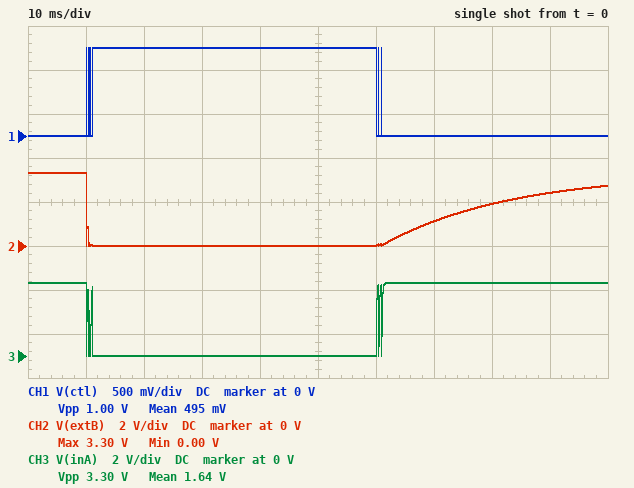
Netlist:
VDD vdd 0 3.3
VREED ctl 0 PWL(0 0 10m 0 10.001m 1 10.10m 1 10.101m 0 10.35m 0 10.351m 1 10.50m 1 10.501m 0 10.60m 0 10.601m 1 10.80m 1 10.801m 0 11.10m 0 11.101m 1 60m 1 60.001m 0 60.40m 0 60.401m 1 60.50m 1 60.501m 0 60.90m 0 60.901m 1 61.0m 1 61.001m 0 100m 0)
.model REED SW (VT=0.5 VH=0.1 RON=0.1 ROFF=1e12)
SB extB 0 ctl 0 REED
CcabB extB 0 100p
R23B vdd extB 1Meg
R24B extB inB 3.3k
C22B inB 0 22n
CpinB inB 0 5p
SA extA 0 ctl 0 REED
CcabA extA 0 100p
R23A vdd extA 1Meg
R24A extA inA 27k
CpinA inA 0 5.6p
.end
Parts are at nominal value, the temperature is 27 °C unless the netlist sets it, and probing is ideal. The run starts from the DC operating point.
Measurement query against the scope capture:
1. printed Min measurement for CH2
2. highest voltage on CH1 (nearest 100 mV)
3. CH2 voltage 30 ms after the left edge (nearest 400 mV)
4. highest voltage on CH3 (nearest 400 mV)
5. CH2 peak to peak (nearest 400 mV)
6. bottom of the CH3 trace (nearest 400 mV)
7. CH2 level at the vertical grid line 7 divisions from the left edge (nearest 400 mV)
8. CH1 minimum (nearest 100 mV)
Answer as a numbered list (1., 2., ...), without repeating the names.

1. 0.00 V
2. 1.0 V
3. 0 V
4. 3.2 V
5. 3.2 V
6. 0 V
7. 1.2 V
8. 0 V
